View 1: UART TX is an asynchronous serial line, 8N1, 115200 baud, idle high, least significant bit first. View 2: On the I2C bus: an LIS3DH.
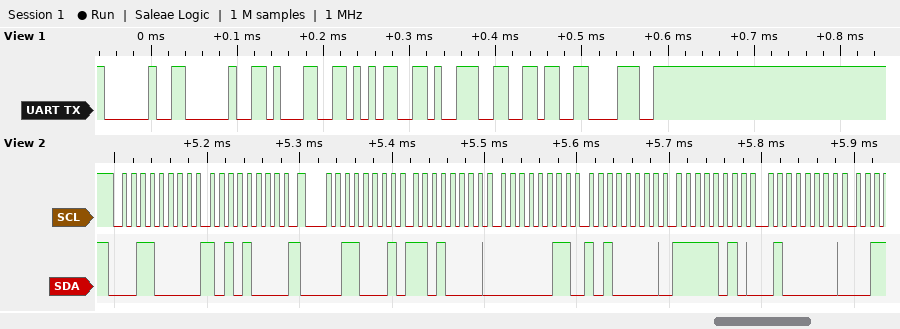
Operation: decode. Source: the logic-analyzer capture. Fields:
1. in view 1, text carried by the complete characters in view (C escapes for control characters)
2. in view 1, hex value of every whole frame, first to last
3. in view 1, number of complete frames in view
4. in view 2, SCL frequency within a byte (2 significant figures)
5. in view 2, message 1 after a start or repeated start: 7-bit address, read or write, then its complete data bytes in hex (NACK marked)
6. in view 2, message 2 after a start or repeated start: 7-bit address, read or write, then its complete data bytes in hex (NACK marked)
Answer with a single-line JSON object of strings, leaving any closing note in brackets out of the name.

{"in view 1, text carried by the complete characters in view": "\"  15968\"", "in view 1, hex value of every whole frame, first to last": "0x20 0x20 0x31 0x35 0x39 0x36 0x38", "in view 1, number of complete frames in view": "7", "in view 2, SCL frequency within a byte": "100 kHz", "in view 2, message 1 after a start or repeated start: 7-bit address, read or write, then its complete data bytes in hex": "0x18 write: A8", "in view 2, message 2 after a start or repeated start: 7-bit address, read or write, then its complete data bytes in hex": "0x18 read: D0 03 A0 FA 40"}
